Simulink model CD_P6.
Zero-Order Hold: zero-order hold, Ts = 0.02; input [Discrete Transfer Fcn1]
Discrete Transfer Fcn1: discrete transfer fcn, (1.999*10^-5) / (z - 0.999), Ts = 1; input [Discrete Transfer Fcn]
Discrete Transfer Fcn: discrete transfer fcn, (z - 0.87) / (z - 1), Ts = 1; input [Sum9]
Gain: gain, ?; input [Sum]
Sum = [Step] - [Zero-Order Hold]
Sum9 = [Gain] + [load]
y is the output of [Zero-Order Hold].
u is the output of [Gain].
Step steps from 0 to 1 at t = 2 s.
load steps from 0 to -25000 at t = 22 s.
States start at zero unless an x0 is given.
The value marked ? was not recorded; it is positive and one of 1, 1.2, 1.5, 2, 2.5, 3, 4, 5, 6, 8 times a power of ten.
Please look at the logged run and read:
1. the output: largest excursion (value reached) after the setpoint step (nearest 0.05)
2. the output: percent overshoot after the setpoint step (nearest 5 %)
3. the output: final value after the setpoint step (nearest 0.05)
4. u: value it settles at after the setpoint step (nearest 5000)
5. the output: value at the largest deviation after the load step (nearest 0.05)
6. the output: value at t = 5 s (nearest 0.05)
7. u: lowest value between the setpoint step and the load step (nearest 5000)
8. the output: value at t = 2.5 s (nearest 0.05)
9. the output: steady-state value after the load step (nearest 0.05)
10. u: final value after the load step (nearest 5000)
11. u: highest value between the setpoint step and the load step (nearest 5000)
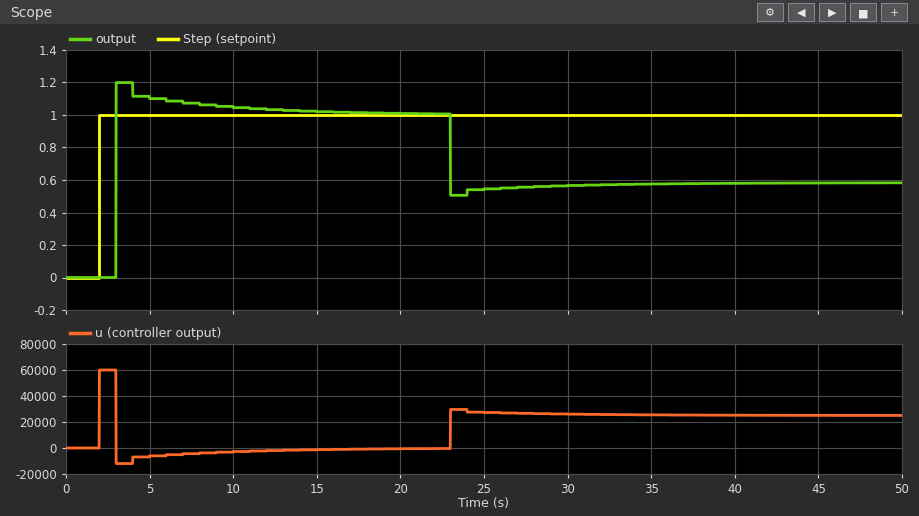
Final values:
1.20
20 %
1.00
0
0.50
1.10
-10000
0.00
0.60
25000
60000
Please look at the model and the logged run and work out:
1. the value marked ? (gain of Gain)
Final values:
60000
